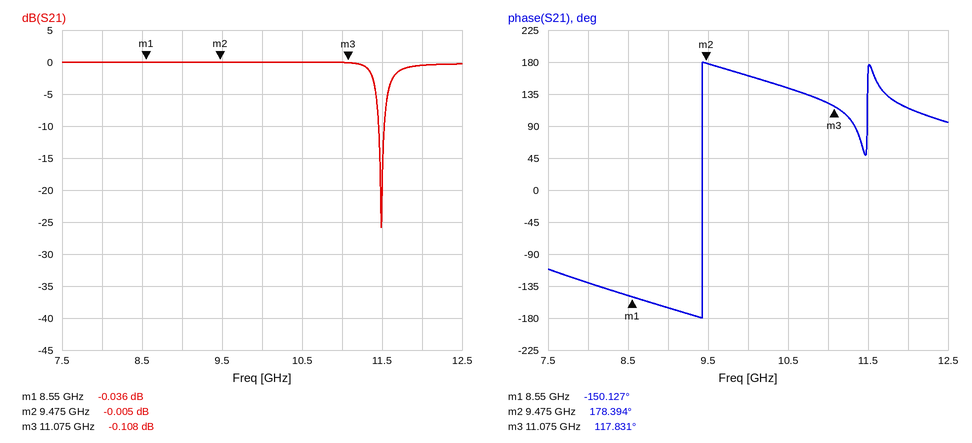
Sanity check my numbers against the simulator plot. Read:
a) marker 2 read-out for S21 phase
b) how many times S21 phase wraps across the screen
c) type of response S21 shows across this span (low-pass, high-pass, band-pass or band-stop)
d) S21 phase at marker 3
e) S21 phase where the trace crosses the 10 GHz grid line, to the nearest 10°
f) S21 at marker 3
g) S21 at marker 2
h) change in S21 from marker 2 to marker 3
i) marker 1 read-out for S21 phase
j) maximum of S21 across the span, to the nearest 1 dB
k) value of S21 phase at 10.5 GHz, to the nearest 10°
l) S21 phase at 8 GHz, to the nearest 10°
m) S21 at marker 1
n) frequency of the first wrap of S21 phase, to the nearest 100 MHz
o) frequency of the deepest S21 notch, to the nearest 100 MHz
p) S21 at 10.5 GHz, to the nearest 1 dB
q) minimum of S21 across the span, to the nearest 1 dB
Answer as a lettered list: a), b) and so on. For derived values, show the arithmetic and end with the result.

a) 178.394°
b) 1
c) band-stop
d) 117.831°
e) 160°
f) -0.108 dB
g) -0.005 dB
h) -0.108 − (-0.005) = -0.103 dB
i) -150.127°
j) 0 dB
k) 140°
l) -130°
m) -0.036 dB
n) 9.4 GHz
o) 11.5 GHz
p) 0 dB
q) -26 dB
